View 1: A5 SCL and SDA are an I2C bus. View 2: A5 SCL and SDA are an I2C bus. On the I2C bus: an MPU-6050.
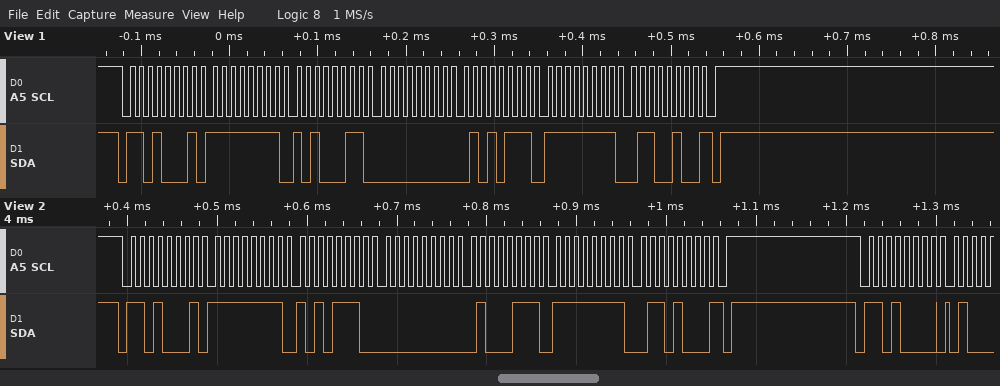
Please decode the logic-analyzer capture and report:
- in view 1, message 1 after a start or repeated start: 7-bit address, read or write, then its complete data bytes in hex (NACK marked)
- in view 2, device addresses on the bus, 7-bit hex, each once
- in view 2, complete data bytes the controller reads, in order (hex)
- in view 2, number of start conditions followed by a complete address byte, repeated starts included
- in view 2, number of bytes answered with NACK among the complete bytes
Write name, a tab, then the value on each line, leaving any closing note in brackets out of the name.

in view 1, message 1 after a start or repeated start: 7-bit address, read or write, then its complete data bytes in hex	0x68 read: FF A3 00 57 FF 64 NACK
in view 2, device addresses on the bus, 7-bit hex, each once	0x68
in view 2, complete data bytes the controller reads, in order	FF AE 00 47 FF 68
in view 2, number of start conditions followed by a complete address byte, repeated starts included	2
in view 2, number of bytes answered with NACK among the complete bytes	1
